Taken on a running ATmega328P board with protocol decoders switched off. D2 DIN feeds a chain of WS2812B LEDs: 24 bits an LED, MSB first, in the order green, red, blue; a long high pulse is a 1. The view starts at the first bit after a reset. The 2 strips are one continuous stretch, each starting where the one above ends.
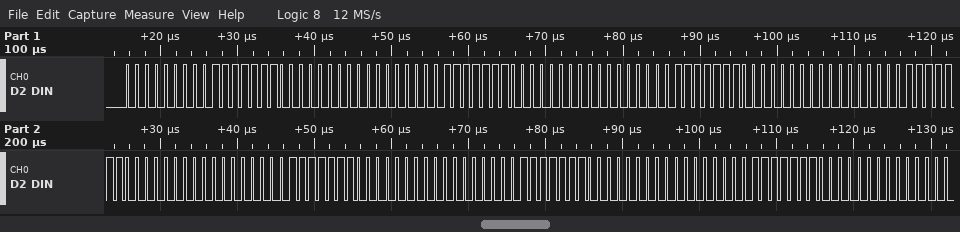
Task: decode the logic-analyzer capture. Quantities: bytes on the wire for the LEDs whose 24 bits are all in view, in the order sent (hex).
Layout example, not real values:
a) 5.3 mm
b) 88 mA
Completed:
a) 00 7F 00 00 7F 00 00 7F 00 00 7F 00 00 7F 00 00 7F 00 00 7F 00
